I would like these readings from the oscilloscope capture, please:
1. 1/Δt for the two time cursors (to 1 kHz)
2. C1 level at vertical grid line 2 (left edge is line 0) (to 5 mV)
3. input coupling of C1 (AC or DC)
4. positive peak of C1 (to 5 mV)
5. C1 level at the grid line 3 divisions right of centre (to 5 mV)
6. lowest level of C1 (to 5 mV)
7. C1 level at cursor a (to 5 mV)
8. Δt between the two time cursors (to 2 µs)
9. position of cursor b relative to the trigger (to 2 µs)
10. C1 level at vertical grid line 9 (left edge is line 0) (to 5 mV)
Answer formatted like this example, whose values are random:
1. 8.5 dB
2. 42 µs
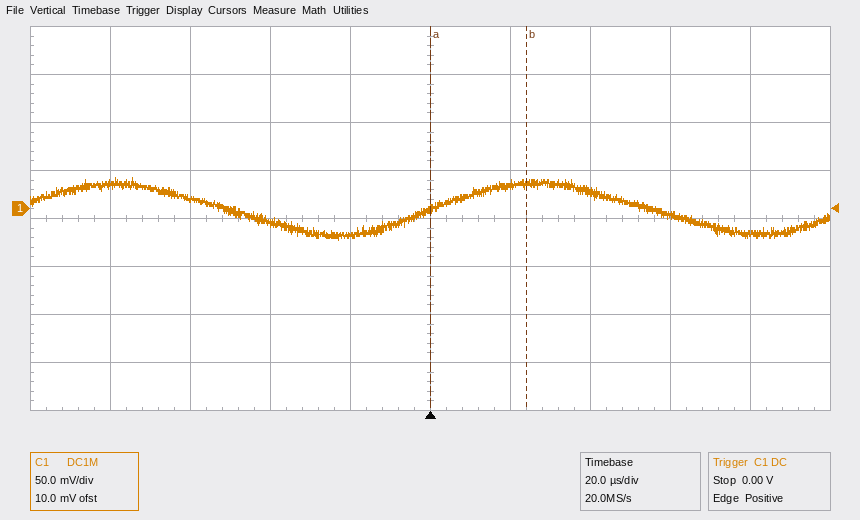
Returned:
1. 42 kHz
2. 10 mV
3. DC
4. 35 mV
5. -5 mV
6. -35 mV
7. 0 mV
8. 24 µs
9. +24 µs
10. -25 mV
